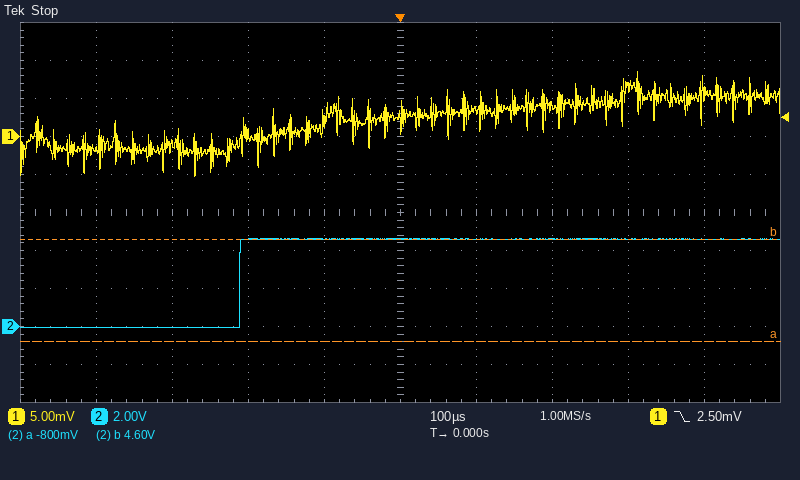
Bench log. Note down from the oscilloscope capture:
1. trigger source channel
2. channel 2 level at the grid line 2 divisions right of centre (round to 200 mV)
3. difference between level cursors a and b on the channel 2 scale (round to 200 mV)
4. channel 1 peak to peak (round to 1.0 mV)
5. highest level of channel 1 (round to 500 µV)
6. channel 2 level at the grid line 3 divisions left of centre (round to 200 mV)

channel 1
4.6 V
5.4 V
14.0 mV
8.5 mV
0.0 V
